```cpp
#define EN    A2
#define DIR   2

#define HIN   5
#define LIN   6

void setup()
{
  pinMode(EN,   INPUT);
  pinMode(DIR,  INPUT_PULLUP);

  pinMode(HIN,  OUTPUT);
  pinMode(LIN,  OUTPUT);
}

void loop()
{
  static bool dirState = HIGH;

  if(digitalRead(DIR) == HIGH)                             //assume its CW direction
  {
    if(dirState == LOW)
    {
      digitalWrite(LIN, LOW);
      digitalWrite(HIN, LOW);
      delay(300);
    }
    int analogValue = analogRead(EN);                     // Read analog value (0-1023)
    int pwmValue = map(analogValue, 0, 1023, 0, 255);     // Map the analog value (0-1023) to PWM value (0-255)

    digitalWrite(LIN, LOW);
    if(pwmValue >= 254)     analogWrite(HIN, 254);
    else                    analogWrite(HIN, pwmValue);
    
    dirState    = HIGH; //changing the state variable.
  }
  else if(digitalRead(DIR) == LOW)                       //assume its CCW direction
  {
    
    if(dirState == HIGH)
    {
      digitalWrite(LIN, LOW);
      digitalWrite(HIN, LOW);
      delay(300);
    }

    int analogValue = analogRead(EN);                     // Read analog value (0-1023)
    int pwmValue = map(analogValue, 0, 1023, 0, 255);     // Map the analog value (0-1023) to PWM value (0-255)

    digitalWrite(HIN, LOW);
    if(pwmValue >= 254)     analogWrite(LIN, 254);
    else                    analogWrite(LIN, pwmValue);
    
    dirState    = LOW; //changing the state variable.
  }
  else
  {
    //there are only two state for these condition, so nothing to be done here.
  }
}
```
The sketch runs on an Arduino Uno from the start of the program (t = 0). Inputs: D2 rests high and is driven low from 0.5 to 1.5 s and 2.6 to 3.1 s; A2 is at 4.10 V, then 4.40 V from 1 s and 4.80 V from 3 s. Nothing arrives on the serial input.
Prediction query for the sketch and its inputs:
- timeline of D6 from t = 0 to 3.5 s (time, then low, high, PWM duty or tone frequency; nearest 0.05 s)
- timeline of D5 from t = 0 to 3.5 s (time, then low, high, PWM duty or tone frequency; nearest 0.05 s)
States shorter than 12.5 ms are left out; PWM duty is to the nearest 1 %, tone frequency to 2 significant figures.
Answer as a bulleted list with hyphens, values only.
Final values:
- 0 s low; 0.8 s PWM 82 %; 1 s PWM 88 %; 1.5 s low; 2.9 s PWM 88 %; 3 s PWM 96 %; 3.1 s low
- 0 s PWM 82 %; 0.5 s low; 1.8 s PWM 88 %; 2.6 s low; 3.4 s PWM 96 %
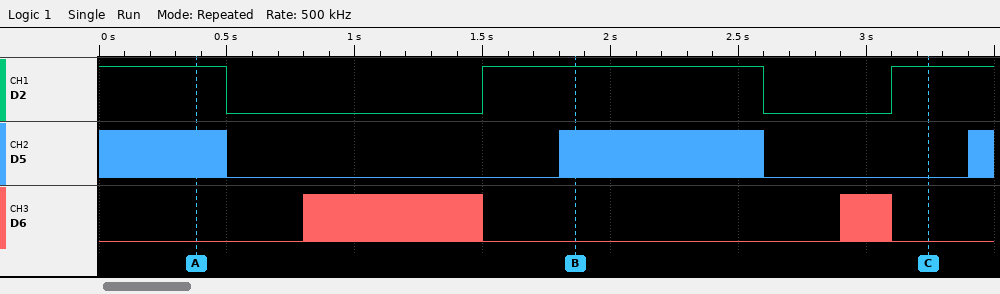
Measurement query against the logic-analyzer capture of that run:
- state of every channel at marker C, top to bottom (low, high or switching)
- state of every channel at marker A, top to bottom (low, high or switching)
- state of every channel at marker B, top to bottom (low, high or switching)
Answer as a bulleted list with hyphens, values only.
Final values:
- D2 high, D5 low, D6 low
- D2 high, D5 switching, D6 low
- D2 high, D5 switching, D6 low
